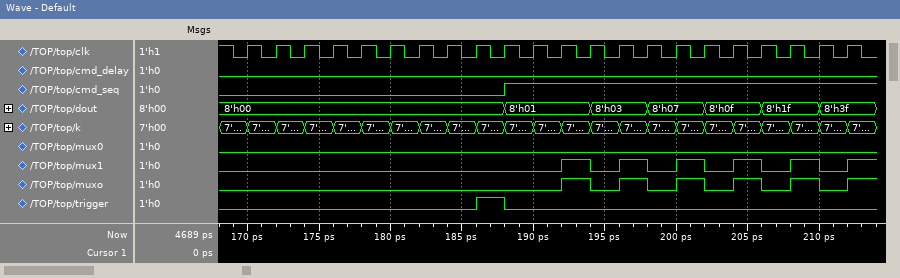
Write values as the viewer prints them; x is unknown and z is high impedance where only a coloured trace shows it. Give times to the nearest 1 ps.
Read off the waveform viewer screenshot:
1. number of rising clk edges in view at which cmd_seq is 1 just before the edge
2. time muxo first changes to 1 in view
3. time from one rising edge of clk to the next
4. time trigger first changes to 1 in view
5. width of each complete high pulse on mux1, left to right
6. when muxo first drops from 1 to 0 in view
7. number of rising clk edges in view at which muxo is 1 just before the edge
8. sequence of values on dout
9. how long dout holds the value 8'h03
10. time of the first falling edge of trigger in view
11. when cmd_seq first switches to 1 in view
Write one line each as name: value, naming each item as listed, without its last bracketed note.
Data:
number of rising clk edges in view at which cmd_seq is 1 just before the edge: 12
time muxo first changes to 1 in view: 192 ps
time from one rising edge of clk to the next: 2 ps
time trigger first changes to 1 in view: 186 ps
width of each complete high pulse on mux1, left to right: 2 ps, 2 ps, 2 ps, 2 ps, 2 ps
when muxo first drops from 1 to 0 in view: 194 ps
number of rising clk edges in view at which muxo is 1 just before the edge: 5
sequence of values on dout: 8'h00, 8'h01, 8'h03, 8'h07, 8'h0f, 8'h1f, 8'h3f
how long dout holds the value 8'h03: 4 ps
time of the first falling edge of trigger in view: 188 ps
when cmd_seq first switches to 1 in view: 188 ps
